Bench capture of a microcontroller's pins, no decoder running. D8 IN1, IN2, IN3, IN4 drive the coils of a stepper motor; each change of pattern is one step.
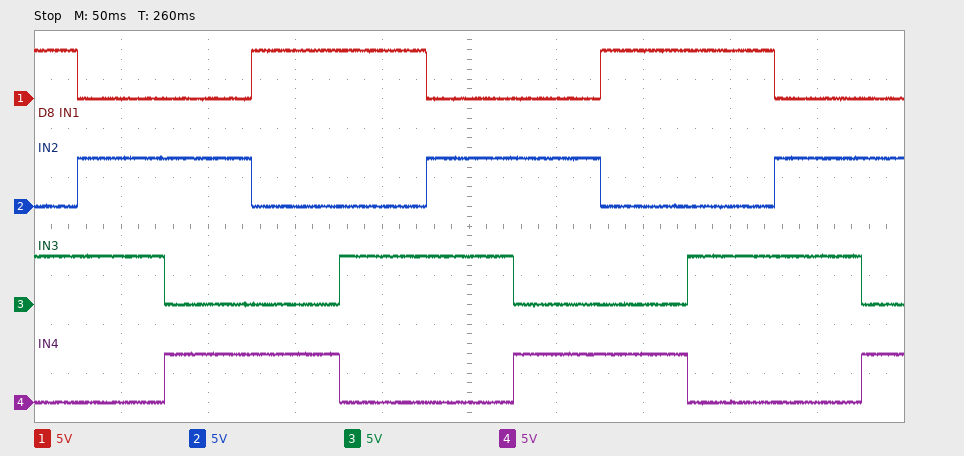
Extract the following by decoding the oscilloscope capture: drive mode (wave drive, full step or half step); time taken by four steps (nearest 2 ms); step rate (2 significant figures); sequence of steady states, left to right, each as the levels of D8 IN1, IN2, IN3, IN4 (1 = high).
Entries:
full step
200 ms
20 steps/s
1010 0110 0101 1001 1010 0110 0101 1001 1010 0110 0101
